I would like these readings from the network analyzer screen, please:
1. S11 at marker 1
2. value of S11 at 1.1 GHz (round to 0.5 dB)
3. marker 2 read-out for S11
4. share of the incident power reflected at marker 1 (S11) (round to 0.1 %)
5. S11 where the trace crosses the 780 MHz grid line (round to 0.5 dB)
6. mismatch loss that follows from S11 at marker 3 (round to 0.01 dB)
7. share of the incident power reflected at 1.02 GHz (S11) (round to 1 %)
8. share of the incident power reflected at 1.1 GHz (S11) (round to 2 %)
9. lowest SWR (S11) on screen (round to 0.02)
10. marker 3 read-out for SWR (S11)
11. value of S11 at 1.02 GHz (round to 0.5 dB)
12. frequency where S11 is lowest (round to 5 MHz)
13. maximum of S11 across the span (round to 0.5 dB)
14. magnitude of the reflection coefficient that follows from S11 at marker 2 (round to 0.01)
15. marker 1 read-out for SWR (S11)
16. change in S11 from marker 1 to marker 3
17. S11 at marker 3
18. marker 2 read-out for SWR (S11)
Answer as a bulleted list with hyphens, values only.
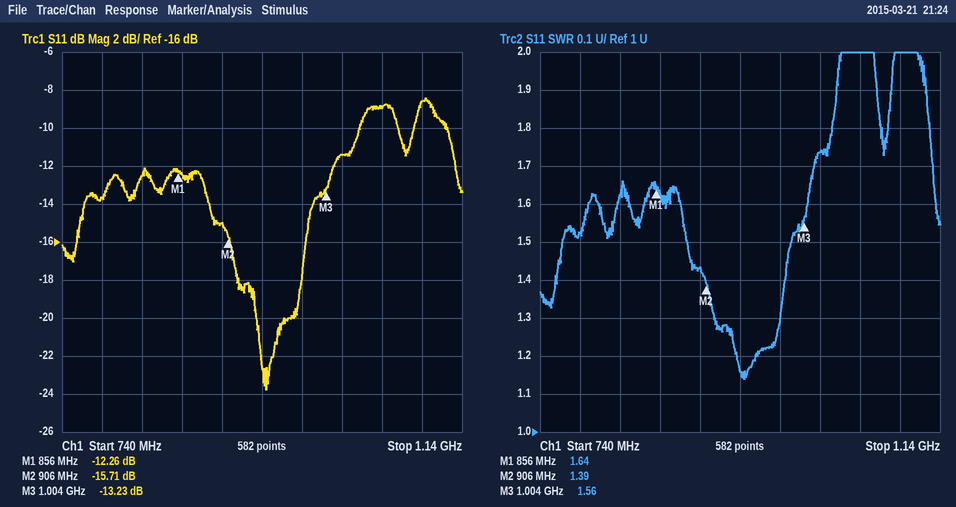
- -12.26 dB
- -8.5 dB
- -15.71 dB
- 5.9 %
- -13.5 dB
- 0.21 dB
- 7 %
- 14 %
- 1.14
- 1.56
- -11.5 dB
- 945 MHz
- -8.5 dB
- 0.16
- 1.64
- -0.97 dB
- -13.23 dB
- 1.39
